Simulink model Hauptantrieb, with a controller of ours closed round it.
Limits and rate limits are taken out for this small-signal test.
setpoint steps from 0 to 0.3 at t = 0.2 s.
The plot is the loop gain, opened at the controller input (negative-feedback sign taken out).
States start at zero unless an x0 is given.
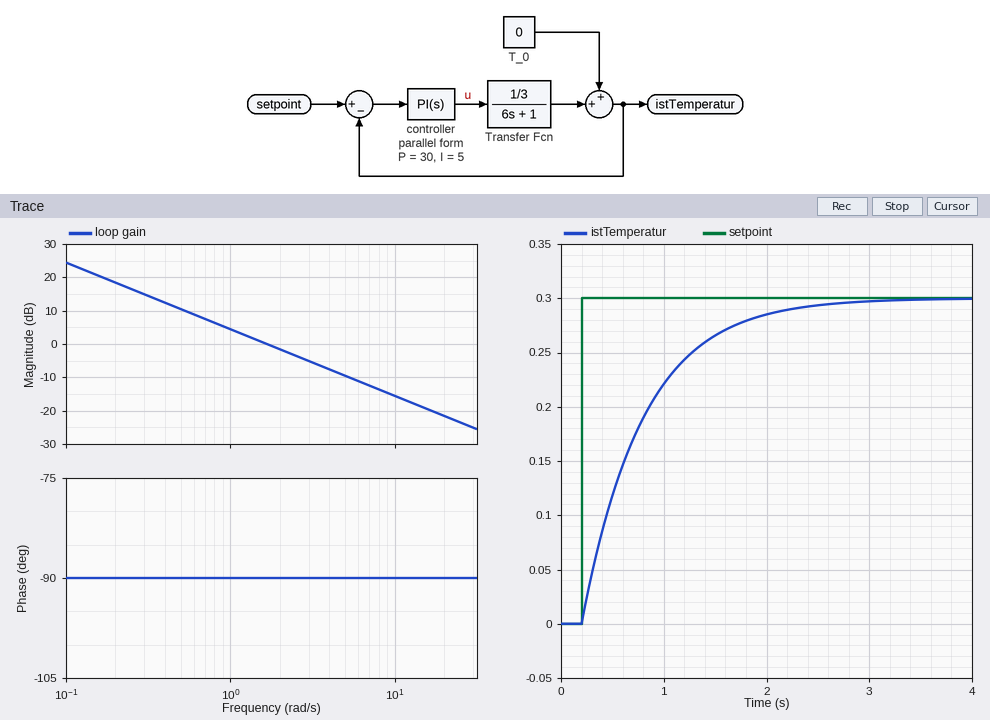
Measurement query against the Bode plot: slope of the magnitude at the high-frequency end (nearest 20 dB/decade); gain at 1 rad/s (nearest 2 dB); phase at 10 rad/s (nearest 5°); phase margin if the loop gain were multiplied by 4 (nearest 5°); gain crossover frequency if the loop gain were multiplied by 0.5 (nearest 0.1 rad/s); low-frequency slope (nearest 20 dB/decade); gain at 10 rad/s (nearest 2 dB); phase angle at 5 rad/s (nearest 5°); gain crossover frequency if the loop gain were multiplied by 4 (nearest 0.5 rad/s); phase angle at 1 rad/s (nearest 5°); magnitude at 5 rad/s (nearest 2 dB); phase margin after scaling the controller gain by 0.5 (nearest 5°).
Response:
-20 dB/decade
4 dB
-90°
90°
0.8 rad/s
-20 dB/decade
-16 dB
-90°
6.5 rad/s
-90°
-10 dB
90°
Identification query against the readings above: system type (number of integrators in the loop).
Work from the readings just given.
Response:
1
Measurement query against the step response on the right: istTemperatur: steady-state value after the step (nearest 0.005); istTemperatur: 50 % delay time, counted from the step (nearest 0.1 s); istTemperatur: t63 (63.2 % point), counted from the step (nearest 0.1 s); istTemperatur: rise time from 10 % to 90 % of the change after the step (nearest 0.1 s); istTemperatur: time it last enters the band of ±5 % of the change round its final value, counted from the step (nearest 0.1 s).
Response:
0.300
0.4 s
0.6 s
1.3 s
1.8 s
